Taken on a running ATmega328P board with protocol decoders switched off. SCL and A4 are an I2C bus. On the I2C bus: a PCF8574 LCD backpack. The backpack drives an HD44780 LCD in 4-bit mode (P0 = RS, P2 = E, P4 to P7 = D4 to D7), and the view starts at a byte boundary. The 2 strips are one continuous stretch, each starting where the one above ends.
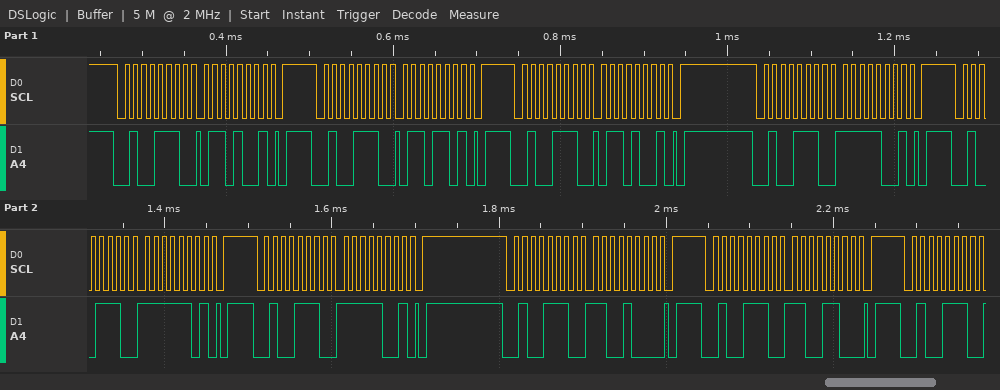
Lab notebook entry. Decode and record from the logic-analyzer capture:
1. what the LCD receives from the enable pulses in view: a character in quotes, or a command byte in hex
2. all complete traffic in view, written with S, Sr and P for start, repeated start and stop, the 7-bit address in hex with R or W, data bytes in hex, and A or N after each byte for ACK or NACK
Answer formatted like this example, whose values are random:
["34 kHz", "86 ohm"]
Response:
["'o'", "S 27W A 69 A P S 27W A 6D A P S 27W A 69 A P S 27W A F9 A P S 27W A FD A P S 27W A F9 A P S 27W A C8 A P S 27W A CC A P S 27W A"]
